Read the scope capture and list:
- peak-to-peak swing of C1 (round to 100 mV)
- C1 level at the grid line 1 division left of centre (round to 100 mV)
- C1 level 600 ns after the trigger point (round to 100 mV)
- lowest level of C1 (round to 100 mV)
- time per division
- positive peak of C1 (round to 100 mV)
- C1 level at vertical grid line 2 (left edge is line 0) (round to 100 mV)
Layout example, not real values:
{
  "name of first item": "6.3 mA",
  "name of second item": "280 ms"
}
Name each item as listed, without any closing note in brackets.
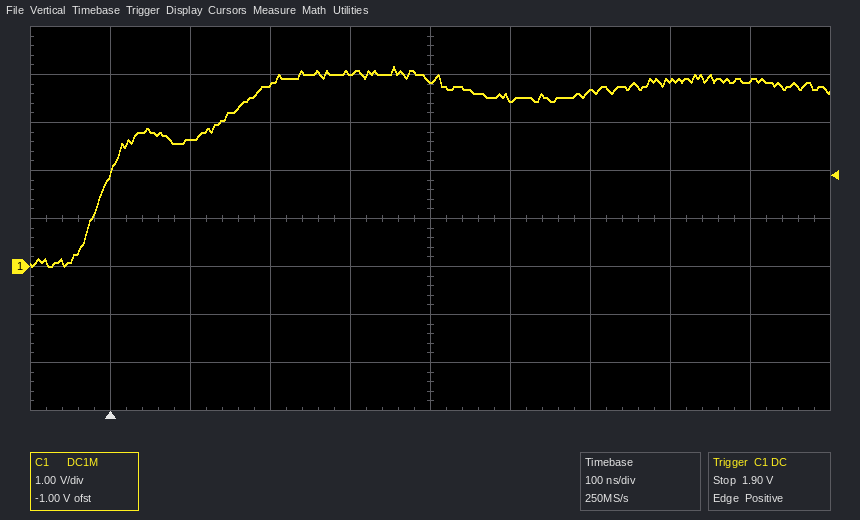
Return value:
{
  "peak-to-peak swing of C1": "4.2 V",
  "C1 level at the grid line 1 division left of centre": "4.0 V",
  "C1 level 600 ns after the trigger point": "3.6 V",
  "lowest level of C1": "0.0 V",
  "time per division": "100 ns",
  "positive peak of C1": "4.2 V",
  "C1 level at vertical grid line 2 (left edge is line 0)": "2.6 V"
}
